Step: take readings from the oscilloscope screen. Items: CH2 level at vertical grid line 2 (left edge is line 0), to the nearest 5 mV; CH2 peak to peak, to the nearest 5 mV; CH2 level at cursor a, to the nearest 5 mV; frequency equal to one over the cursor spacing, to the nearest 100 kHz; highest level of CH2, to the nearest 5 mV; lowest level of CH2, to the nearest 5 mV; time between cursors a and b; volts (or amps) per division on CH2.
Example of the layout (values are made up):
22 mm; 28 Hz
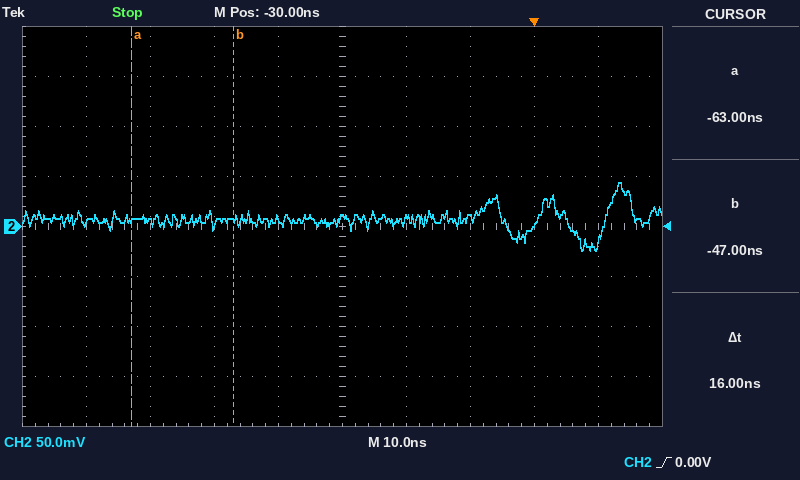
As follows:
5 mV; 70 mV; 5 mV; 62.5 MHz; 45 mV; -25 mV; 16 ns; 50 mV
